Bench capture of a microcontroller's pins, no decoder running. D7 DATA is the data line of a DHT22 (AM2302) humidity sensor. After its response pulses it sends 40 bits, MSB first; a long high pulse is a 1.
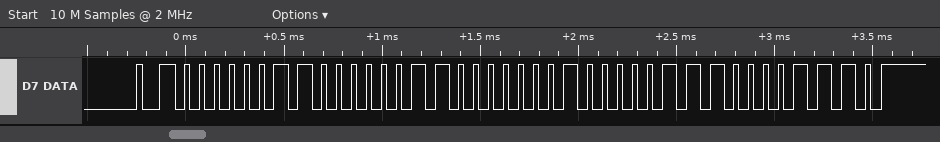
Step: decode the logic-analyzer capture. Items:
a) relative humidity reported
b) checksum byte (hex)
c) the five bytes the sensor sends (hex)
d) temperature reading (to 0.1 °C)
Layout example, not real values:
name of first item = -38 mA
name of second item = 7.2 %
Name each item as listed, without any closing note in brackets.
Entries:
relative humidity reported = 77.1 %
checksum byte = 0x0E
the five bytes the sensor sends = 03 03 01 07 0E
temperature reading = 26.3 °C
